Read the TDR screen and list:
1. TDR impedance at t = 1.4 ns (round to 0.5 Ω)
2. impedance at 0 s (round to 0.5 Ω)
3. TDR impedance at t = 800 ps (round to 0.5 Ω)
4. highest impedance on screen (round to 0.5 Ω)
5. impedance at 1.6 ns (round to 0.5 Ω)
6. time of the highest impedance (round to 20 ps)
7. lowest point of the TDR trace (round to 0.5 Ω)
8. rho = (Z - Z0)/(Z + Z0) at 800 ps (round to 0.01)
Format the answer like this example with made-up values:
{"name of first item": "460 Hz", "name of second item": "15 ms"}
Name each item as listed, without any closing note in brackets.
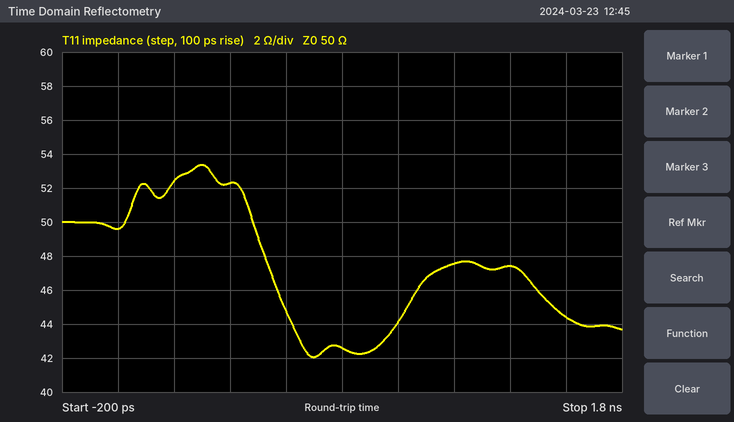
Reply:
{"TDR impedance at t = 1.4 ns": "47.5 Ω", "impedance at 0 s": "49.5 Ω", "TDR impedance at t = 800 ps": "42.5 Ω", "highest impedance on screen": "53.5 Ω", "impedance at 1.6 ns": "44.5 Ω", "time of the highest impedance": "300 ps", "lowest point of the TDR trace": "42.0 Ω", "rho = (Z - Z0)/(Z + Z0) at 800 ps": "-0.08"}
